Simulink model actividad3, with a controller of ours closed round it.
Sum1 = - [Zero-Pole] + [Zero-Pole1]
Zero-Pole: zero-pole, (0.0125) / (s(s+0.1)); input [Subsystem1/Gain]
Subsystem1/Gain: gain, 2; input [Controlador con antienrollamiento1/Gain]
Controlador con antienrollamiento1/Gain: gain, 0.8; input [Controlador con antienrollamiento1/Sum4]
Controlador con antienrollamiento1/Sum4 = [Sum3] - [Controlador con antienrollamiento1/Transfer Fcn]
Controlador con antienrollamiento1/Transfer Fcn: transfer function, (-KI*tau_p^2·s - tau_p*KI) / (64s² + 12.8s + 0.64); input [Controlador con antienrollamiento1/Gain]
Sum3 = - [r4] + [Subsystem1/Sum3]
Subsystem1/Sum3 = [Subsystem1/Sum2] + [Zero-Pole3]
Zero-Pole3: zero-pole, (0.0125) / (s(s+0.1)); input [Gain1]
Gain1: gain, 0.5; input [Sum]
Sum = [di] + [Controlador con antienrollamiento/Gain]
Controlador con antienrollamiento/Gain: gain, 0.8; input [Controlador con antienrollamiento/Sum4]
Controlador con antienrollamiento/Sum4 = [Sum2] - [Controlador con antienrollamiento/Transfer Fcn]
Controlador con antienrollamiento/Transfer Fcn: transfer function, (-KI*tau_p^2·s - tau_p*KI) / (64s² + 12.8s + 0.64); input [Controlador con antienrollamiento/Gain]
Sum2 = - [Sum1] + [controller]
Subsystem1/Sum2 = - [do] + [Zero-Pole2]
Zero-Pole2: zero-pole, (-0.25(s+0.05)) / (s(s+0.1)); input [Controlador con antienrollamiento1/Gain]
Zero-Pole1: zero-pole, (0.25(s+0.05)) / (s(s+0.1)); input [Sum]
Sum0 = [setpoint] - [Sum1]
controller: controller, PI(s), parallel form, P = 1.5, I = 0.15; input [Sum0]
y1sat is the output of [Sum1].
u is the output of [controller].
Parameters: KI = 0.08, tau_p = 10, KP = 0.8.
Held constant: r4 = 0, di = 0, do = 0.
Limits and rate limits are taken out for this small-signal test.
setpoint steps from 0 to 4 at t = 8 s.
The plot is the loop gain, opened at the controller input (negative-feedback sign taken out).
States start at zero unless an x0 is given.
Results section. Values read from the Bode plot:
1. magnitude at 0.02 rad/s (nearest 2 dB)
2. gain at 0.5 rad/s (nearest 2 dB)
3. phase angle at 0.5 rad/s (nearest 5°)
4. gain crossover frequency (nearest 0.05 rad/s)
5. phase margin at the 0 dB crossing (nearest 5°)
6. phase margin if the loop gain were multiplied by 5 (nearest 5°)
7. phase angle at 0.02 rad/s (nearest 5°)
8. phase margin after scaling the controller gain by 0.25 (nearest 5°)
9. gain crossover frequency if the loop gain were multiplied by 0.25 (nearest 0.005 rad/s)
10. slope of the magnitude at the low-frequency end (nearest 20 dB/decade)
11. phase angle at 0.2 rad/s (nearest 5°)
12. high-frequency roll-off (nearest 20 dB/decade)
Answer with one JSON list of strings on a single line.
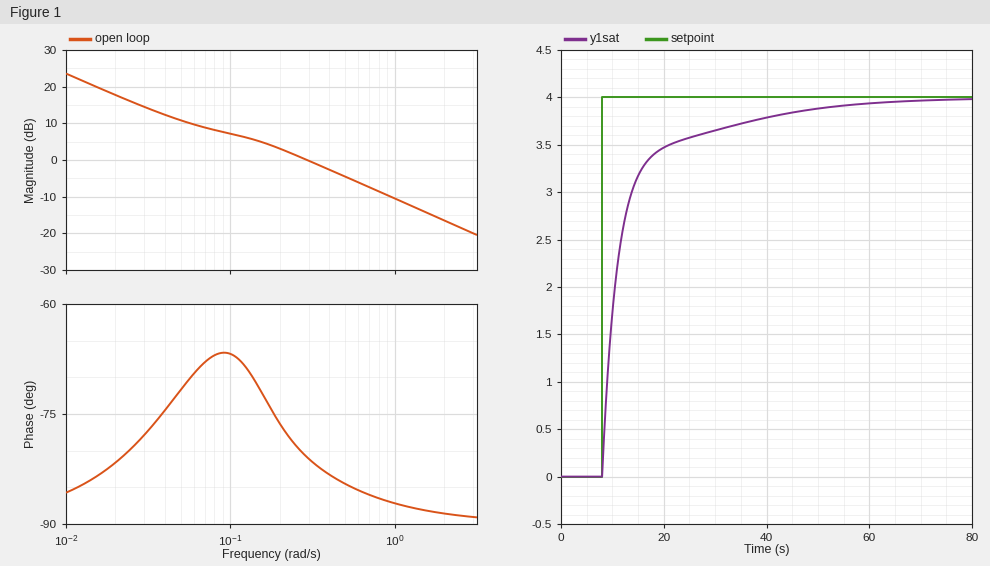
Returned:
["18 dB", "-4 dB", "-85°", "0.30 rad/s", "100°", "90°", "-80°", "105°", "0.040 rad/s", "-20 dB/decade", "-75°", "-20 dB/decade"]
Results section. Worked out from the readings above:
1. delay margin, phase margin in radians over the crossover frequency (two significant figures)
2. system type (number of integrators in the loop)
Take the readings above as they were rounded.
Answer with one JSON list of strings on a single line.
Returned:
["5.8 s", "1"]
